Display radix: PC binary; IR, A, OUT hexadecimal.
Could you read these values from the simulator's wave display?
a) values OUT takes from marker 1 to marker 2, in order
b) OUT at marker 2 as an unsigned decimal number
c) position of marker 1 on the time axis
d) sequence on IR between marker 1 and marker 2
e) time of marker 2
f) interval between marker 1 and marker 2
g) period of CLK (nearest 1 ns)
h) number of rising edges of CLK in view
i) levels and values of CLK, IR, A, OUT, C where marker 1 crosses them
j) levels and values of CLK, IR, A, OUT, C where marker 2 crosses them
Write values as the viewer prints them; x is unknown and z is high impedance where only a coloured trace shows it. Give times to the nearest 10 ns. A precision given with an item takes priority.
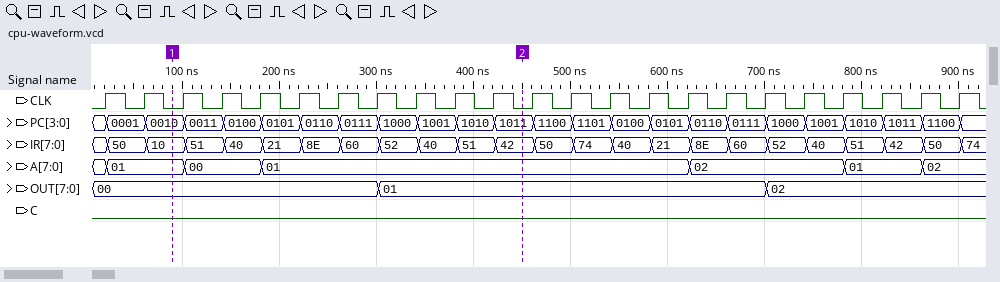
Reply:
00, 01
1
90 ns
10, 51, 40, 21, 8E, 60, 52, 40, 51, 42
450 ns
360 ns
40 ns
23
CLK=0, IR=10, A=01, OUT=00, C=0
CLK=0, IR=42, A=01, OUT=01, C=0
